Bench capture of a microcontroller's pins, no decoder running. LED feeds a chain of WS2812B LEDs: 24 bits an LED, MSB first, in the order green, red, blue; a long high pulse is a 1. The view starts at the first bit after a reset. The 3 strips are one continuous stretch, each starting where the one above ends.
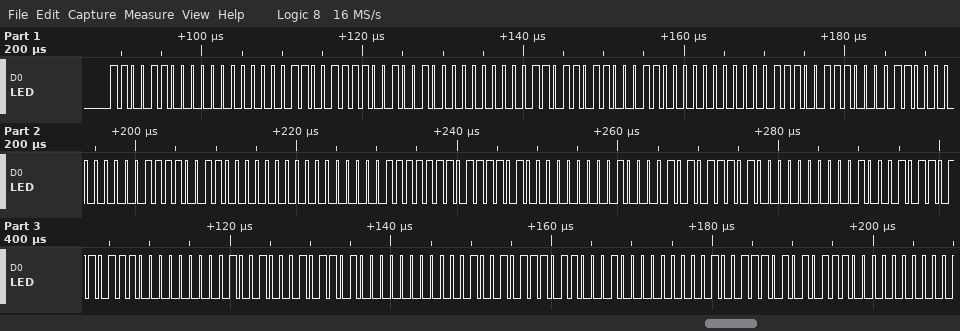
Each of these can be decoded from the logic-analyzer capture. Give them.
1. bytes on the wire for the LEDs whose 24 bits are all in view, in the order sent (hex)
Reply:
CC 00 33 C9 00 36 C6 00 39 C3 00 3C C0 00 3F BD 00 42 BA 00 45 B7 00 48 B4 00 4B B1 00 4E
